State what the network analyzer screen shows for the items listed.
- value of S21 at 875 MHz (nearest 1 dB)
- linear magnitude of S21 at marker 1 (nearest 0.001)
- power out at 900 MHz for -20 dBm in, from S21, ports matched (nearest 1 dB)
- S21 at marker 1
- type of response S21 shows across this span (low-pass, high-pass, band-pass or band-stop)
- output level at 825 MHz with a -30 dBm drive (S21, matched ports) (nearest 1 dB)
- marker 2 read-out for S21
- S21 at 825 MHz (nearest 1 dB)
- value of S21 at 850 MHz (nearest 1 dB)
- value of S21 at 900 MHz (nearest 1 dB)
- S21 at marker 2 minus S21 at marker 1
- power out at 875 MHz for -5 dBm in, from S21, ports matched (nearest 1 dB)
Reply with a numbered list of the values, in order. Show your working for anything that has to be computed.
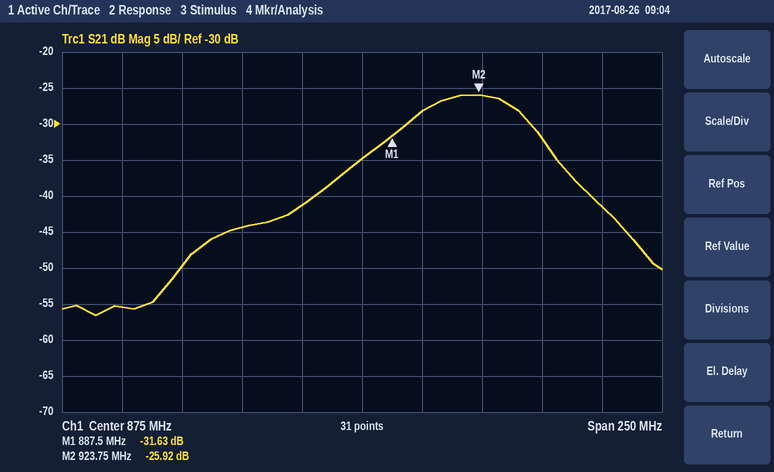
1. -35 dB
2. 10^(-31.63/20) ≈ 0.026
3. -20 dBm + (-28 dB) = -48 dBm
4. -31.63 dB
5. band-pass
6. -30 dBm + (-44 dB) = -74 dBm
7. -25.92 dB
8. -44 dB
9. -41 dB
10. -28 dB
11. -25.92 − (-31.63) = 5.71 dB
12. -5 dBm + (-35 dB) = -40 dBm
